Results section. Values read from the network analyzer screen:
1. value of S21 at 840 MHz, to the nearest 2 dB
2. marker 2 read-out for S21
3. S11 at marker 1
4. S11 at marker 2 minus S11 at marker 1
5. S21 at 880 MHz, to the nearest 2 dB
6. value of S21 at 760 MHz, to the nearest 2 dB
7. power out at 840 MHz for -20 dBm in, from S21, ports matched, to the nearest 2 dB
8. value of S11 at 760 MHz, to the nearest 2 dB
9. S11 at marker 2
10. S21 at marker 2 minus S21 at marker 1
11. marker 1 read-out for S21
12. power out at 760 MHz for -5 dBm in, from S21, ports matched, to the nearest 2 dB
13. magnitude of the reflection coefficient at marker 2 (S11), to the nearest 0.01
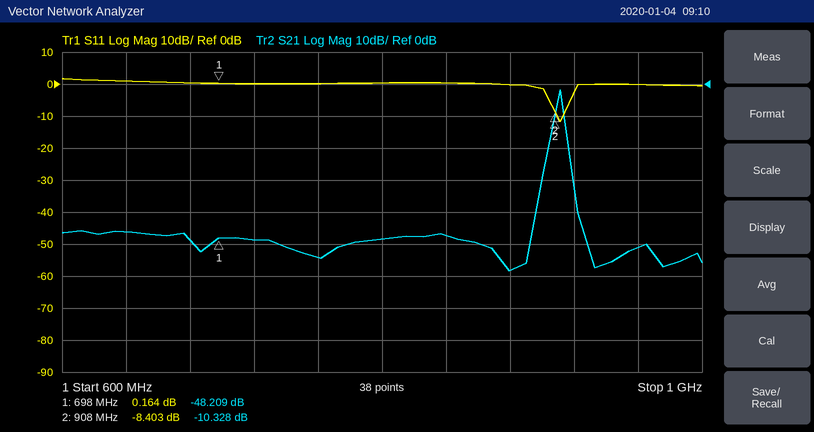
-48 dB
-10.328 dB
0.164 dB
-8.567 dB
-58 dB
-54 dB
-68 dBm
0 dB
-8.403 dB
37.881 dB
-48.209 dB
-60 dBm
0.38
